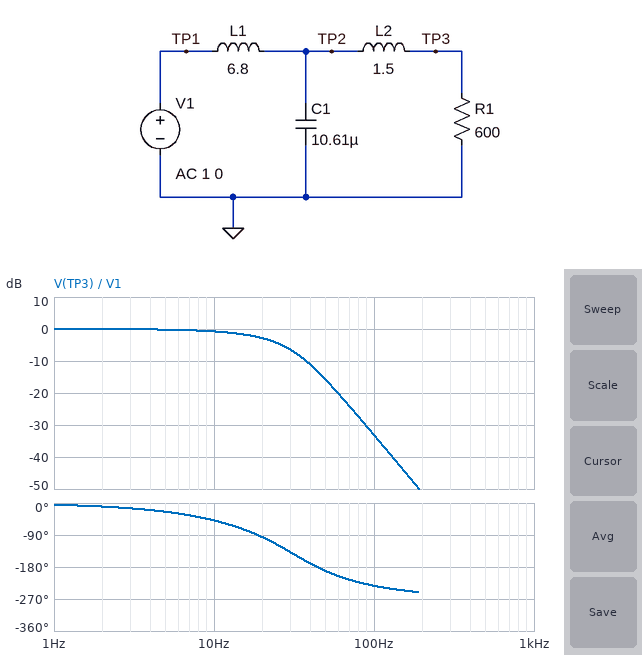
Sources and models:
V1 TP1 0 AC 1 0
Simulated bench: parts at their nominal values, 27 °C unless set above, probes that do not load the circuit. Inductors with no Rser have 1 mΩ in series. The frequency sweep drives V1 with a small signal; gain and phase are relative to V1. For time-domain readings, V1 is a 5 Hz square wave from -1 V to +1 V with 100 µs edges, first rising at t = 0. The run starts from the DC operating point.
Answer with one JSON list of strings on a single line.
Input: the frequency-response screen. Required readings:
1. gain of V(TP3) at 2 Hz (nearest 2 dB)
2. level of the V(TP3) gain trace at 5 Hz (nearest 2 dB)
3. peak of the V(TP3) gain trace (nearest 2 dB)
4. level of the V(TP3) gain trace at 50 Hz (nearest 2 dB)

["0 dB", "0 dB", "0 dB", "-16 dB"]
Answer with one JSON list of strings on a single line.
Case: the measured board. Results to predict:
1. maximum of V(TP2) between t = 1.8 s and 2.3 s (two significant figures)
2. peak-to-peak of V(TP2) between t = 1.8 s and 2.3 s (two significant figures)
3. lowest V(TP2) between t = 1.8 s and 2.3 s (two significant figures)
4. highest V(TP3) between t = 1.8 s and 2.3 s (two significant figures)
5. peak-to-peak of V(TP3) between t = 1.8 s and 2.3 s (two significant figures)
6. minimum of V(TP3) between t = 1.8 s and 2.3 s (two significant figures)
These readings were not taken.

["1.0 V", "2.0 V", "-1.0 V", "1.0 V", "2.0 V", "-1.0 V"]
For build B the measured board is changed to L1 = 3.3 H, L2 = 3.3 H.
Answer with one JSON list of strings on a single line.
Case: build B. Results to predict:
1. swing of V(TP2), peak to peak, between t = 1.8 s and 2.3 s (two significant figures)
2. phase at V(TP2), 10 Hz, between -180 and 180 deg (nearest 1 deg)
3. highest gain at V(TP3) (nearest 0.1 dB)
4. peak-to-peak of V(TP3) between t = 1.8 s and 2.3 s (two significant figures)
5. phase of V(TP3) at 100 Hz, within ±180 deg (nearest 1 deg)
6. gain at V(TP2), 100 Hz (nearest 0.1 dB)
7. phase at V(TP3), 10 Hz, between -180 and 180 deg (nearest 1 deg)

["3.2 V", "-18 deg", "2.4 dB", "2.5 V", "107 deg", "-21.5 dB", "-37 deg"]
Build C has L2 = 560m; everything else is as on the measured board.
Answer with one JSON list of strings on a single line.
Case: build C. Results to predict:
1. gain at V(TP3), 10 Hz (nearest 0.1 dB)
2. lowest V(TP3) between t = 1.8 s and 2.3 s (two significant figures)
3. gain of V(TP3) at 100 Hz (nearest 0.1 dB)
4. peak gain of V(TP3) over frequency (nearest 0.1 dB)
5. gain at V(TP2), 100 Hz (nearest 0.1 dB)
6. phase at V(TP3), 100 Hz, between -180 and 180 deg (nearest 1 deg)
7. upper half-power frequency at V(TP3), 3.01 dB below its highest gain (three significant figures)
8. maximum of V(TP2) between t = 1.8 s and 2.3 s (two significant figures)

["-0.3 dB", "-1.1 V", "-29.2 dB", "0 dB", "-27.9 dB", "162 deg", "20.0 Hz", "1.1 V"]
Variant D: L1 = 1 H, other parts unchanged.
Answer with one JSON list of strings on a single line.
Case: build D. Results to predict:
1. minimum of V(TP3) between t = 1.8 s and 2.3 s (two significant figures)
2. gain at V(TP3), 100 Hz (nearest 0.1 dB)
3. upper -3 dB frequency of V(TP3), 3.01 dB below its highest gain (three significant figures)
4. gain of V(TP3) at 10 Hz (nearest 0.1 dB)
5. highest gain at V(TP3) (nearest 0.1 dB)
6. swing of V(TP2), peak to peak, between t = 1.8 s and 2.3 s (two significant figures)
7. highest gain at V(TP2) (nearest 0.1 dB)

["-1.7 V", "-14.1 dB", "62.1 Hz", "0.1 dB", "7.2 dB", "4.1 V", "9.6 dB"]
